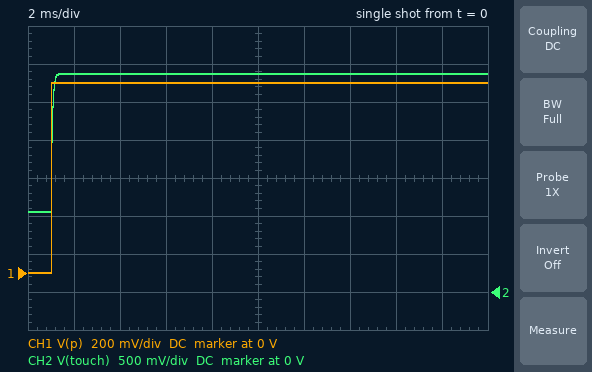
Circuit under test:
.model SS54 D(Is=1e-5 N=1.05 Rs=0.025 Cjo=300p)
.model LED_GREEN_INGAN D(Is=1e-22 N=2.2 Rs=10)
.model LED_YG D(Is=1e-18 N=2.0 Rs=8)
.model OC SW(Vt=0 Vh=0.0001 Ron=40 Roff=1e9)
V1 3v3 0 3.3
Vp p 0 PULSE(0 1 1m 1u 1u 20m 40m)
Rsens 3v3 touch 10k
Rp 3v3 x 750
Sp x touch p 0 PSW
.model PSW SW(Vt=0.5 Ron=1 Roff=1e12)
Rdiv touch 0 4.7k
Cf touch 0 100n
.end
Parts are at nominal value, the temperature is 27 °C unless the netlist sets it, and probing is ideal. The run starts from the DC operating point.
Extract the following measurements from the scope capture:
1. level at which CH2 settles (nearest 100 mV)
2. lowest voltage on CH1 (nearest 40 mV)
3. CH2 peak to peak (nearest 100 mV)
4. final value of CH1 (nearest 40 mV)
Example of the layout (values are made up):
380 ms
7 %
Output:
2.9 V
0 V
1.8 V
1.00 V
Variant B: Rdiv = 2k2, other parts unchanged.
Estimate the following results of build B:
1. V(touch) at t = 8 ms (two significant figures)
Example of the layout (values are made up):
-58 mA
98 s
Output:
2.5 V
